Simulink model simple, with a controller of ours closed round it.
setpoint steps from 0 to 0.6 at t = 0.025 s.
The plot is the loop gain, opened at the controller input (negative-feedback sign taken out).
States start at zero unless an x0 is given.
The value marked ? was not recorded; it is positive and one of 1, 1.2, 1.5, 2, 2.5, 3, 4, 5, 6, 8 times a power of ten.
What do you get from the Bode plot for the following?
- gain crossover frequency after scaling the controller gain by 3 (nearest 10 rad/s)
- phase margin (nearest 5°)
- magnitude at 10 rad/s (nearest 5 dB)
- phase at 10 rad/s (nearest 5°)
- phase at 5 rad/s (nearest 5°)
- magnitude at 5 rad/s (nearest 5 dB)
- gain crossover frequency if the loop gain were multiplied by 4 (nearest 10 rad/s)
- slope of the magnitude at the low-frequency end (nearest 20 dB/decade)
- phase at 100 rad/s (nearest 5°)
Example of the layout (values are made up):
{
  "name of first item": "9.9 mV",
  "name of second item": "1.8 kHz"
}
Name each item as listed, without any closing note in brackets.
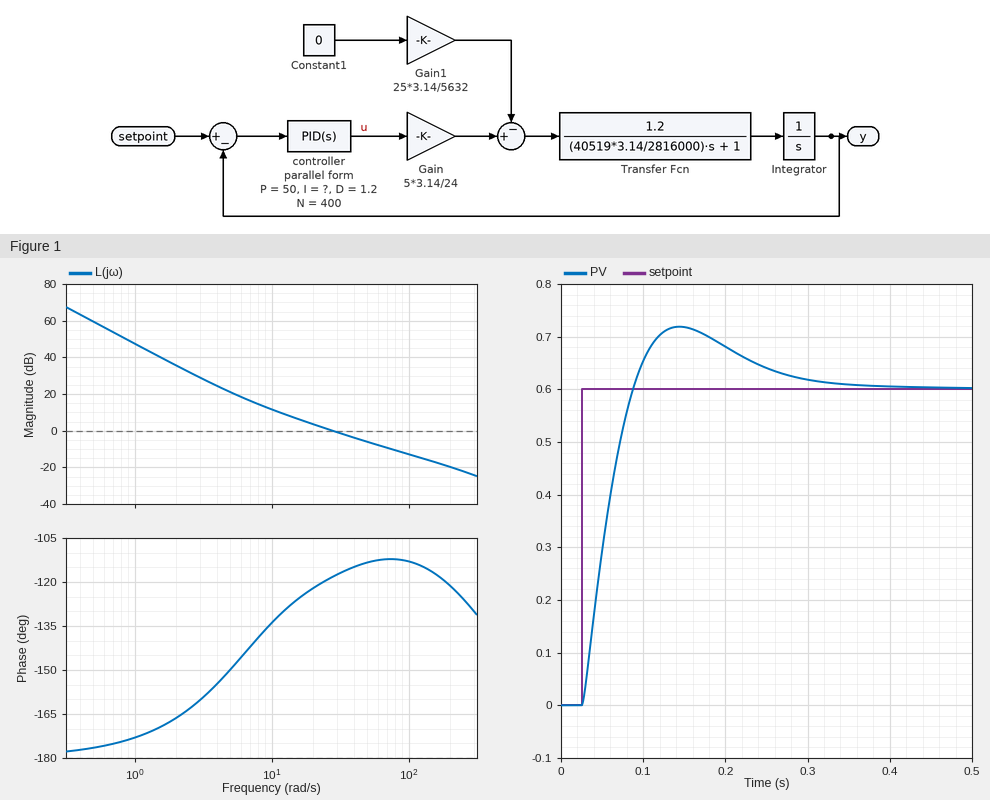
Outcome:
{
  "gain crossover frequency after scaling the controller gain by 3": "70 rad/s",
  "phase margin": "60°",
  "magnitude at 10 rad/s": "10 dB",
  "phase at 10 rad/s": "-135°",
  "phase at 5 rad/s": "-150°",
  "magnitude at 5 rad/s": "20 dB",
  "gain crossover frequency if the loop gain were multiplied by 4": "90 rad/s",
  "slope of the magnitude at the low-frequency end": "-40 dB/decade",
  "phase at 100 rad/s": "-115°"
}
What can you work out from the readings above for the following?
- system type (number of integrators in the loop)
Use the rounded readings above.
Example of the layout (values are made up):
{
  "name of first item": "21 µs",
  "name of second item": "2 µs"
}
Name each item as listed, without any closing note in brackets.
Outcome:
{
  "system type": "2"
}
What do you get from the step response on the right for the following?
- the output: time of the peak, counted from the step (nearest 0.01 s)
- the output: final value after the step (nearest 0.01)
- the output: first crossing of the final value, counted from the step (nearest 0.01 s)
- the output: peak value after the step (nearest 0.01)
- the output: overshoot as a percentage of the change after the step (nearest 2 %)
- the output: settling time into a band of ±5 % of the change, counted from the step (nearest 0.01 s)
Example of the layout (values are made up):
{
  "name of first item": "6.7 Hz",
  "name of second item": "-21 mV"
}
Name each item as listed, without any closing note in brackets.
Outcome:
{
  "the output: time of the peak, counted from the step": "0.12 s",
  "the output: final value after the step": "0.60",
  "the output: first crossing of the final value, counted from the step": "0.06 s",
  "the output: peak value after the step": "0.72",
  "the output: overshoot as a percentage of the change after the step": "20 %",
  "the output: settling time into a band of ±5 % of the change, counted from the step": "0.24 s"
}
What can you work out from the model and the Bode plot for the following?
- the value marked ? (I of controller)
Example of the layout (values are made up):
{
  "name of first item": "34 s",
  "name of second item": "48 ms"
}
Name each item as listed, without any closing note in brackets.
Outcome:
{
  "the value marked ?": "300"
}
